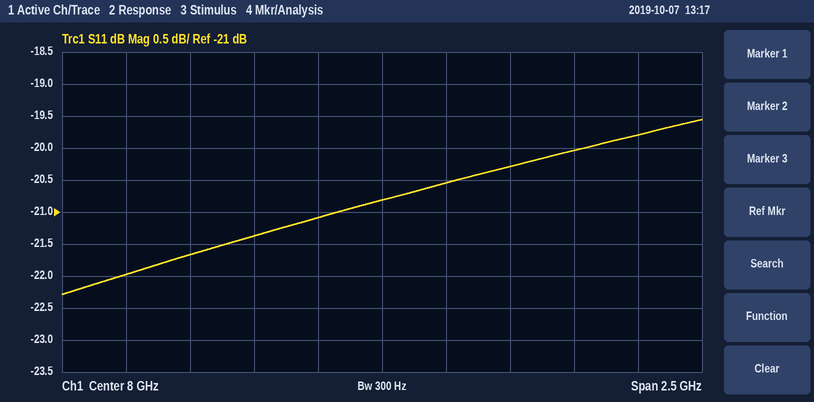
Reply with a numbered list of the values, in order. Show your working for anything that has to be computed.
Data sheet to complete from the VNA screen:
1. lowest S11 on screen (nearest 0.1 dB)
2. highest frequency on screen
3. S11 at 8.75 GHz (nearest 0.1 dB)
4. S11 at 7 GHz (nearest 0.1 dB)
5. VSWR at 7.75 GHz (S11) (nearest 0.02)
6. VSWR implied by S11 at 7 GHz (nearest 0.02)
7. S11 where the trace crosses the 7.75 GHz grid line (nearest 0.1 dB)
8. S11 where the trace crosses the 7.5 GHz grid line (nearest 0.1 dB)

1. -22.3 dB
2. 9.25 GHz
3. -20.0 dB
4. -22.0 dB
5. |Γ| = 10^(-21.1/20) = 0.0881; VSWR = (1 + 0.0881)/(1 − 0.0881) ≈ 1.19, so 1.20 to the nearest 0.02
6. |Γ| = 10^(-22/20) = 0.0794; VSWR = (1 + 0.0794)/(1 − 0.0794) ≈ 1.17, so 1.18 to the nearest 0.02
7. -21.1 dB
8. -21.4 dB
